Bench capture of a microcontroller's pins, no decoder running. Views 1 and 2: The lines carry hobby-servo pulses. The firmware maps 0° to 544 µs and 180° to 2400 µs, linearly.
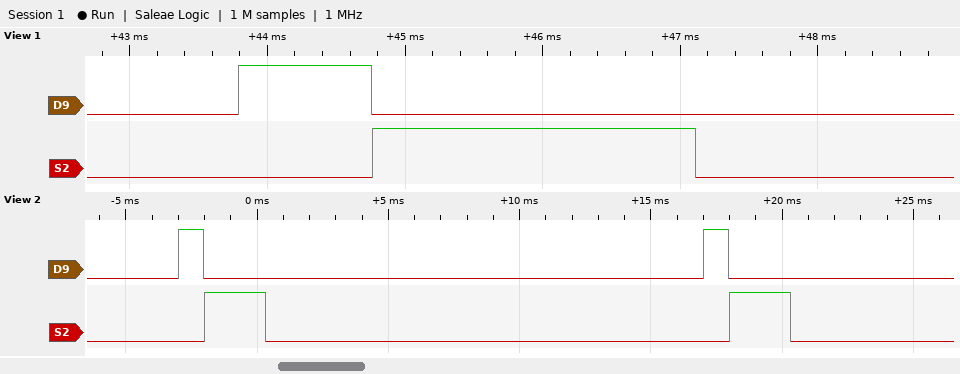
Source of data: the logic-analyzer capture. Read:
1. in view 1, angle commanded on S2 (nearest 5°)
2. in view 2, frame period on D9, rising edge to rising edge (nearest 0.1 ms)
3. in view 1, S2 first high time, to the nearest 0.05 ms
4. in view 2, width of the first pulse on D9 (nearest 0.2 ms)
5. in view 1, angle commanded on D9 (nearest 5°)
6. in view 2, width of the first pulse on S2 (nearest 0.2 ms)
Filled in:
175°
20.0 ms
2.35 ms
1.0 ms
40°
2.4 ms
